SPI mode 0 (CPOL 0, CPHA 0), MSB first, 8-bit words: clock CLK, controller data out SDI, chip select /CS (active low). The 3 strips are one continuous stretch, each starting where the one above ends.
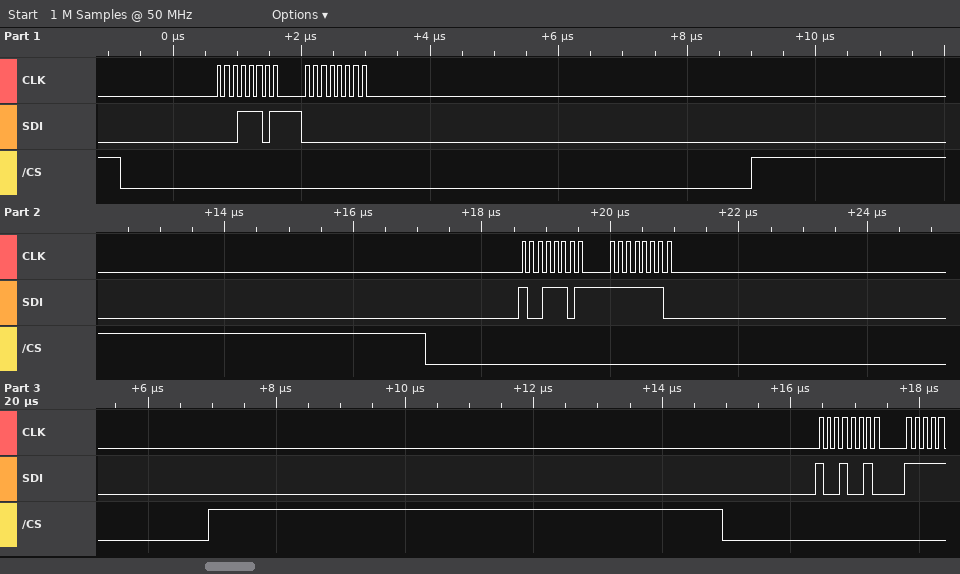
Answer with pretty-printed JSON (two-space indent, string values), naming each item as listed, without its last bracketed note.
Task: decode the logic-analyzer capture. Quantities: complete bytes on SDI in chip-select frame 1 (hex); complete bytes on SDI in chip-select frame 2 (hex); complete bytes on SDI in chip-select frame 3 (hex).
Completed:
{
  "complete bytes on SDI in chip-select frame 1": "1D 00",
  "complete bytes on SDI in chip-select frame 2": "9D FE",
  "complete bytes on SDI in chip-select frame 3": "92"
}
